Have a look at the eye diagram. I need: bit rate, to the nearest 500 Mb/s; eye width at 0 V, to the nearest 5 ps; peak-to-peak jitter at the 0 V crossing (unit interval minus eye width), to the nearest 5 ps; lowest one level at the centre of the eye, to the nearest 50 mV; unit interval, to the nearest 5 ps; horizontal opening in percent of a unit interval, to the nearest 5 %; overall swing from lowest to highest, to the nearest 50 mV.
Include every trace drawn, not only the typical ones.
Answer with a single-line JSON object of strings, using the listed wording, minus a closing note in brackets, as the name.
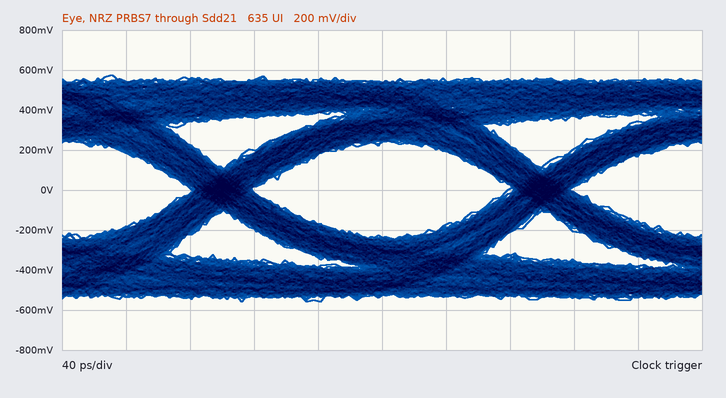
{"bit rate, to the nearest 500 Mb/s": "5.0 Gb/s", "eye width at 0 V, to the nearest 5 ps": "160 ps", "peak-to-peak jitter at the 0 V crossing (unit interval minus eye width), to the nearest 5 ps": "40 ps", "lowest one level at the centre of the eye, to the nearest 50 mV": "250 mV", "unit interval, to the nearest 5 ps": "200 ps", "horizontal opening in percent of a unit interval, to the nearest 5 %": "80 %", "overall swing from lowest to highest, to the nearest 50 mV": "1.15 V"}
